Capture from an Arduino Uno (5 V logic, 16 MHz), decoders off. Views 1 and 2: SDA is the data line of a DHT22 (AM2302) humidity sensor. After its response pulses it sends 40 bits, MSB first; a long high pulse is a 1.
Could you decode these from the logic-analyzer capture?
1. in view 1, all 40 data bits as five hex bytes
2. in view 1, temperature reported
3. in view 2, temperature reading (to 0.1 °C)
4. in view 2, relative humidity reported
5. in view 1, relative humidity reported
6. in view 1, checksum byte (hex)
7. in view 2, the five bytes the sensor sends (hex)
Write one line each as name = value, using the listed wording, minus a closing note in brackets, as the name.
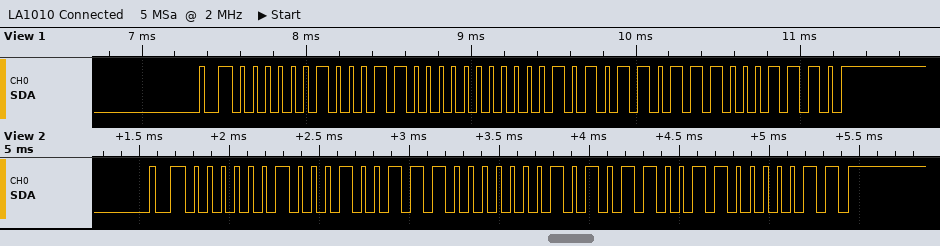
in view 1, all 40 data bits as five hex bytes = 02 30 01 5B 8E
in view 1, temperature reported = 34.7 °C
in view 2, temperature reading = 34.5 °C
in view 2, relative humidity reported = 55.1 %
in view 1, relative humidity reported = 56.0 %
in view 1, checksum byte = 0x8E
in view 2, the five bytes the sensor sends = 02 27 01 59 83
